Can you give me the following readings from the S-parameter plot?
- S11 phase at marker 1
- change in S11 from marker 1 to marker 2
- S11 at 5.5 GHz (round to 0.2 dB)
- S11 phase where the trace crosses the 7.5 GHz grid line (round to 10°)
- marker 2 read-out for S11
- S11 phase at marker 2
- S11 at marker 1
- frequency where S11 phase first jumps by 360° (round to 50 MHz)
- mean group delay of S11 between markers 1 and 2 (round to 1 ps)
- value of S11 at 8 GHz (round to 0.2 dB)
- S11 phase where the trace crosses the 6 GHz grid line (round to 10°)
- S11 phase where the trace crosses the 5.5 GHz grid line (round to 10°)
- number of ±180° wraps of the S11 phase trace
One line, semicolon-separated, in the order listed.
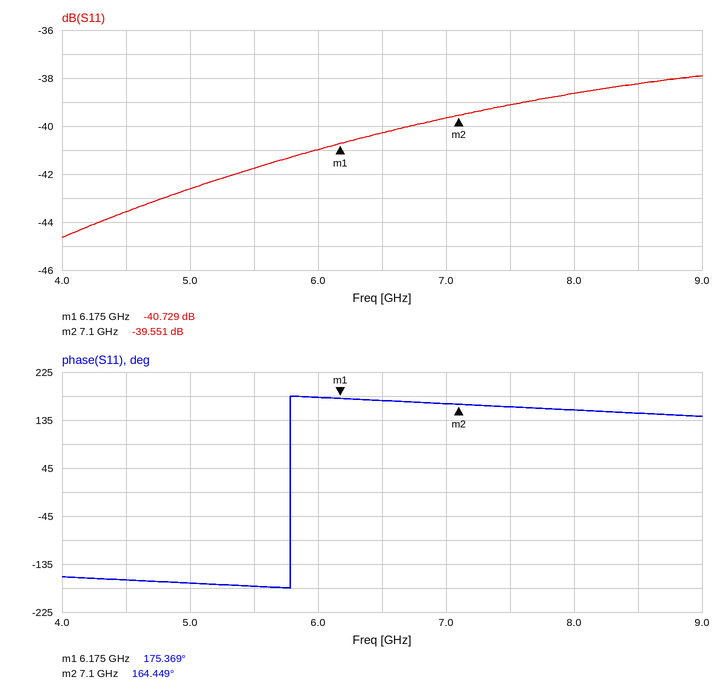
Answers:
175.369°; 1.178 dB; -41.8 dB; 160°; -39.551 dB; 164.449°; -40.729 dB; 5.80 GHz; 33 ps; -38.6 dB; 180°; -180°; 1
